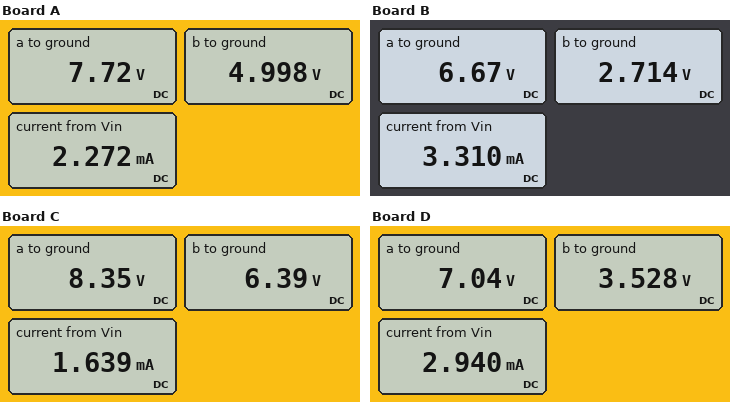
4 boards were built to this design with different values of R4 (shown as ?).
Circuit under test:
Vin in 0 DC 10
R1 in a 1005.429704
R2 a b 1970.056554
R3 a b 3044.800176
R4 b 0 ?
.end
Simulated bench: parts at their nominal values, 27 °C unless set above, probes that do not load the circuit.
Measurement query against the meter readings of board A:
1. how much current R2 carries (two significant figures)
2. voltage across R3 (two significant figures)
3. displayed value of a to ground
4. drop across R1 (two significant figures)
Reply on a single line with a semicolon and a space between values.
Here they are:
1.4 mA; 2.7 V; 7.72 V; 2.3 V
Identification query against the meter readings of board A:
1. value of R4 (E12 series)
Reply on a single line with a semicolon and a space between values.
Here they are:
2.2 kΩ
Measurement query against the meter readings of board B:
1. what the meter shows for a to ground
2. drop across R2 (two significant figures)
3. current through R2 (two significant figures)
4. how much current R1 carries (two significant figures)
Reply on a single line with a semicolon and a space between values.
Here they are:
6.67 V; 4.0 V; 2.0 mA; 3.3 mA
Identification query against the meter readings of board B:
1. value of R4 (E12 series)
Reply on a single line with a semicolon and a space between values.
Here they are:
820 Ω
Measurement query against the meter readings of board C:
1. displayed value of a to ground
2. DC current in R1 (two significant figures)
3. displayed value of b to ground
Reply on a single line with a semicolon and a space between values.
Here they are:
8.35 V; 1.6 mA; 6.39 V
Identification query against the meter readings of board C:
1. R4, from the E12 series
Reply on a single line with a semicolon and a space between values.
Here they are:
3.9 kΩ
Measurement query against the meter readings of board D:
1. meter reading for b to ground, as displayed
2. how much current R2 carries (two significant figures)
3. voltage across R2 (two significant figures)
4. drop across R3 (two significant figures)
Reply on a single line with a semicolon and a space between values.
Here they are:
3.528 V; 1.8 mA; 3.5 V; 3.5 V
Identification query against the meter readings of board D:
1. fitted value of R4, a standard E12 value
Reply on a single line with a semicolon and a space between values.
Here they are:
1.2 kΩ
